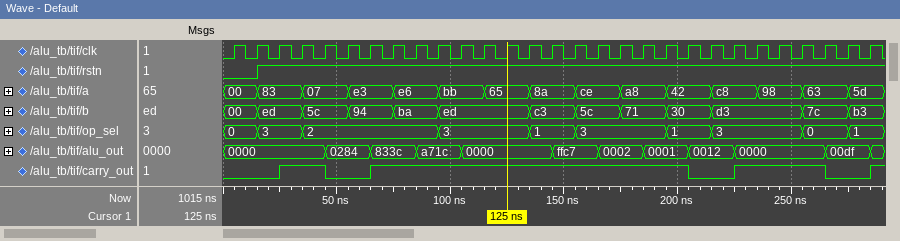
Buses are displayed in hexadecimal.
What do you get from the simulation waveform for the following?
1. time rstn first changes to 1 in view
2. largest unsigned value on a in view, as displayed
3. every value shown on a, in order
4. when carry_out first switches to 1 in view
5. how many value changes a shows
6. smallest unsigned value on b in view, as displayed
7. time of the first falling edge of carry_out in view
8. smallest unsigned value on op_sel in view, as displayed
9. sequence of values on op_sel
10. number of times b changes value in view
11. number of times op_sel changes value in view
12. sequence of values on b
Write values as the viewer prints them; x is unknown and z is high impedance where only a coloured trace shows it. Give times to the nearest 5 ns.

15 ns
e6
00, 83, 07, e3, e6, bb, 65, 8a, ce, a8, 42, c8, 98, 63, 5d
25 ns
14
00
45 ns
0
0, 3, 2, 3, 1, 3, 1, 3, 0, 1
12
9
00, ed, 5c, 94, ba, ed, c3, 5c, 71, 30, d3, 7c, b3
